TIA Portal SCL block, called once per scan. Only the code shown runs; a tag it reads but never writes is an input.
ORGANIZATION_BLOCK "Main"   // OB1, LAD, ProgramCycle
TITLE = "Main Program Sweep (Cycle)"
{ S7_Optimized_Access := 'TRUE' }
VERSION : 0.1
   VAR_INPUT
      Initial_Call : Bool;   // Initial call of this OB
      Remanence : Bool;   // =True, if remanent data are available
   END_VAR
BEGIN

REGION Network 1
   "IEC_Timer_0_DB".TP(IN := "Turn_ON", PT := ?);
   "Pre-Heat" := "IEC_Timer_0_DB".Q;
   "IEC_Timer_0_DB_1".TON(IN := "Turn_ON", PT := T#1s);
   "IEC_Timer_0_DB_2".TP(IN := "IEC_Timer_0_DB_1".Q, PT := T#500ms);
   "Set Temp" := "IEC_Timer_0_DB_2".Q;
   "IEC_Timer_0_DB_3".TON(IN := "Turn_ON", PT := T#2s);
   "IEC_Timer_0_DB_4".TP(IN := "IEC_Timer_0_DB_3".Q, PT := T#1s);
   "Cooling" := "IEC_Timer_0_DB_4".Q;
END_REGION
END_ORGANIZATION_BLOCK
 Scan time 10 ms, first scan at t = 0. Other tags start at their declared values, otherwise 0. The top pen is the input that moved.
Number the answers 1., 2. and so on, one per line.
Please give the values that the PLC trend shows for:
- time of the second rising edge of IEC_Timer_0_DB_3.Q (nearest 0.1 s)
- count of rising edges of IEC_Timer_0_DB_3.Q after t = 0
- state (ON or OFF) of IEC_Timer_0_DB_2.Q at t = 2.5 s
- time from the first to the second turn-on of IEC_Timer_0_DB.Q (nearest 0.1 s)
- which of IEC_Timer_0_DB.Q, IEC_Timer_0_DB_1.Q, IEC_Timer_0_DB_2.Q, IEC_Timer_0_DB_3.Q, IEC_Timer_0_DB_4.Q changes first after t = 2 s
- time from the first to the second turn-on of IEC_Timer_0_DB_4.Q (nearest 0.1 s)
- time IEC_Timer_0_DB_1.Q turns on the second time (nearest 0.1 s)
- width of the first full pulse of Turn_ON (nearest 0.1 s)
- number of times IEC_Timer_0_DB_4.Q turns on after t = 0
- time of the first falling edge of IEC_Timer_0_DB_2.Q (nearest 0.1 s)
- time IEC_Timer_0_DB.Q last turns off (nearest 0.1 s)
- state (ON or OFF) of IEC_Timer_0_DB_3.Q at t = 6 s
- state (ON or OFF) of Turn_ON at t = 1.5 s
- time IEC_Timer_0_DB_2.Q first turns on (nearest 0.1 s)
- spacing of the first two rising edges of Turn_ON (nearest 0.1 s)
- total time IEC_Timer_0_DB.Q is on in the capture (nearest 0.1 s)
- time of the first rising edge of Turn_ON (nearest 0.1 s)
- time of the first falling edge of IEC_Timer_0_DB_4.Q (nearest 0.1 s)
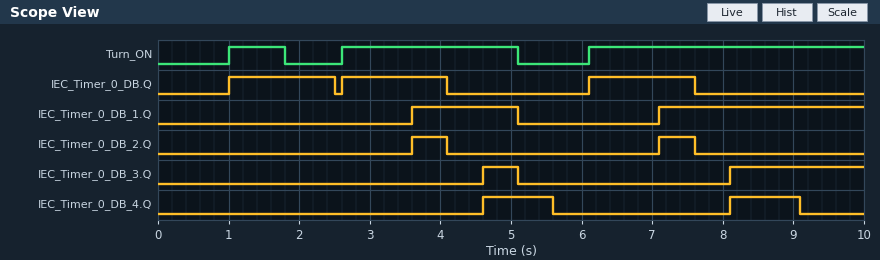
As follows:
1. 8.1 s
2. 2
3. OFF
4. 1.6 s
5. IEC_Timer_0_DB.Q
6. 3.5 s
7. 7.1 s
8. 0.8 s
9. 2
10. 4.1 s
11. 7.6 s
12. OFF
13. ON
14. 3.6 s
15. 1.6 s
16. 4.5 s
17. 1.0 s
18. 5.6 s
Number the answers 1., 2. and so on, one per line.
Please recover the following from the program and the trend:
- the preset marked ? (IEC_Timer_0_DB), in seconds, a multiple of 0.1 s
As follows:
1. 1.5 s
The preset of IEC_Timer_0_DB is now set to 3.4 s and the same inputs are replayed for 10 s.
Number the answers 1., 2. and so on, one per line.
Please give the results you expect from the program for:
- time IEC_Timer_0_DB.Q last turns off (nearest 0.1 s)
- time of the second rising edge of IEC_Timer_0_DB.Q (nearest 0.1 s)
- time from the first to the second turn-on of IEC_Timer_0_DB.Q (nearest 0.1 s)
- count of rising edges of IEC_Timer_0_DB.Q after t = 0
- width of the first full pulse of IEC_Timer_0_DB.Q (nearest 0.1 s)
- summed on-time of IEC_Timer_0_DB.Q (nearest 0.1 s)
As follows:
1. 9.5 s
2. 6.1 s
3. 5.1 s
4. 2
5. 3.4 s
6. 6.8 s
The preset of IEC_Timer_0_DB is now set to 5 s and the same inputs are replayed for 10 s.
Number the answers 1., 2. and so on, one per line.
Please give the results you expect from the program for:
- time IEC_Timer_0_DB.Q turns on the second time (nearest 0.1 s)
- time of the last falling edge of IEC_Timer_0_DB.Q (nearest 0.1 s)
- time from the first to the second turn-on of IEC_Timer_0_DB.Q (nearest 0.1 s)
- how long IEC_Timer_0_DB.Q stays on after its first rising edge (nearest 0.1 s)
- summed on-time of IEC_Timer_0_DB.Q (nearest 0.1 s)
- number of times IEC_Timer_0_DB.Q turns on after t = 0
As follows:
1. 6.1 s
2. 6.0 s
3. 5.1 s
4. 5.0 s
5. 8.9 s
6. 2
